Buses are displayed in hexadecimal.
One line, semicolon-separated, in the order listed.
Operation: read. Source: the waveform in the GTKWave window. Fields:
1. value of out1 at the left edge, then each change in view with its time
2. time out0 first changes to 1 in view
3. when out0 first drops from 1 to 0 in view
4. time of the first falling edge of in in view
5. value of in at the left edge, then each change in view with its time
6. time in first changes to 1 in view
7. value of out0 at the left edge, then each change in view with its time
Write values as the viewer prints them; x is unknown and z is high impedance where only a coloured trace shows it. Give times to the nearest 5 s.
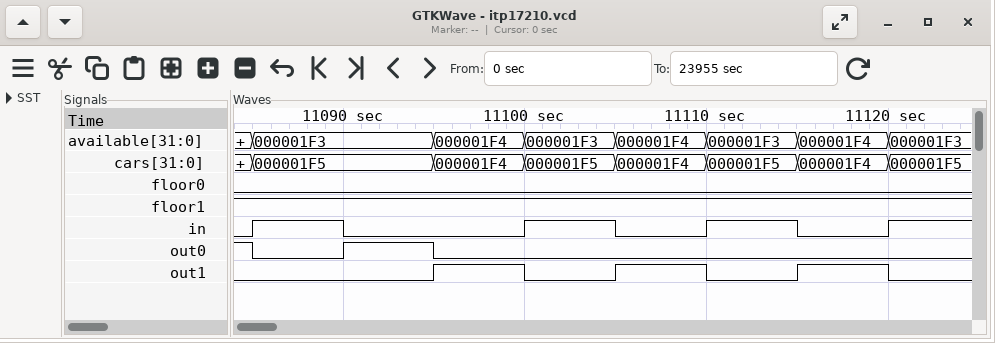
0, 1 at 11095 s, 0 at 11100 s, 1 at 11105 s, 0 at 11110 s, 1 at 11115 s, 0 at 11120 s; 11090 s; 11085 s; 11090 s; 0, 1 at 11085 s, 0 at 11090 s, 1 at 11100 s, 0 at 11105 s, 1 at 11110 s, 0 at 11115 s, 1 at 11120 s; 11085 s; 1, 0 at 11085 s, 1 at 11090 s, 0 at 11095 s
